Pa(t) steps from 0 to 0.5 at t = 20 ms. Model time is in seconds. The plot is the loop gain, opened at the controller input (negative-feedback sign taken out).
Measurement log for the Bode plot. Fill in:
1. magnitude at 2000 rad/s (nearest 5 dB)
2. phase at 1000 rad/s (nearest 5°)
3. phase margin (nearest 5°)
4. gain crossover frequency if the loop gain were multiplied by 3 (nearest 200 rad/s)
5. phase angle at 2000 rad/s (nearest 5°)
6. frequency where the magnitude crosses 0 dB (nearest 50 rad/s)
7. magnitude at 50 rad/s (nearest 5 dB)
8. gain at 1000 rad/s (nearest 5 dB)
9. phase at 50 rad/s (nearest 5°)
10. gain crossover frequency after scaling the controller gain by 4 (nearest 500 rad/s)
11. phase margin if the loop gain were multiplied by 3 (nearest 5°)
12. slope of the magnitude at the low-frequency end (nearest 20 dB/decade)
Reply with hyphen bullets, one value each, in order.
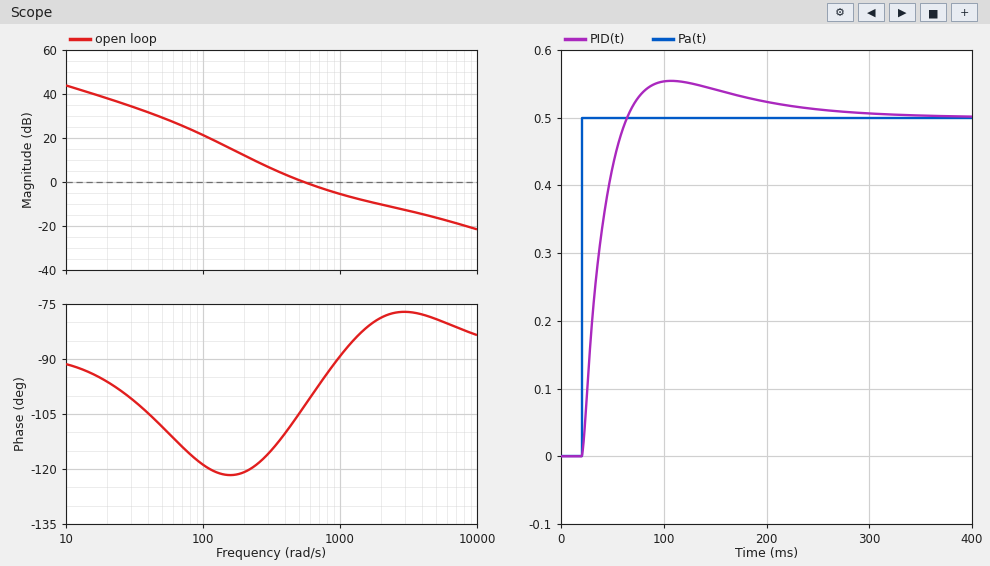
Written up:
- -10 dB
- -90°
- 75°
- 1800 rad/s
- -80°
- 550 rad/s
- 30 dB
- -5 dB
- -110°
- 2500 rad/s
- 100°
- -20 dB/decade
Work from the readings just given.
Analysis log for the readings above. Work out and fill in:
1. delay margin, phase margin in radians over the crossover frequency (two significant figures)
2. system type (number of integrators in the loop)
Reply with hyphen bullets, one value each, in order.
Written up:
- 0.0024 s
- 1
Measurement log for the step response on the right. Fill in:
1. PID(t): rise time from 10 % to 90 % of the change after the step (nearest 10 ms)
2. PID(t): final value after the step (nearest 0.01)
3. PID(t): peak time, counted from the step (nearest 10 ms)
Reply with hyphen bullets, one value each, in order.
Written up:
- 30 ms
- 0.50
- 90 ms
